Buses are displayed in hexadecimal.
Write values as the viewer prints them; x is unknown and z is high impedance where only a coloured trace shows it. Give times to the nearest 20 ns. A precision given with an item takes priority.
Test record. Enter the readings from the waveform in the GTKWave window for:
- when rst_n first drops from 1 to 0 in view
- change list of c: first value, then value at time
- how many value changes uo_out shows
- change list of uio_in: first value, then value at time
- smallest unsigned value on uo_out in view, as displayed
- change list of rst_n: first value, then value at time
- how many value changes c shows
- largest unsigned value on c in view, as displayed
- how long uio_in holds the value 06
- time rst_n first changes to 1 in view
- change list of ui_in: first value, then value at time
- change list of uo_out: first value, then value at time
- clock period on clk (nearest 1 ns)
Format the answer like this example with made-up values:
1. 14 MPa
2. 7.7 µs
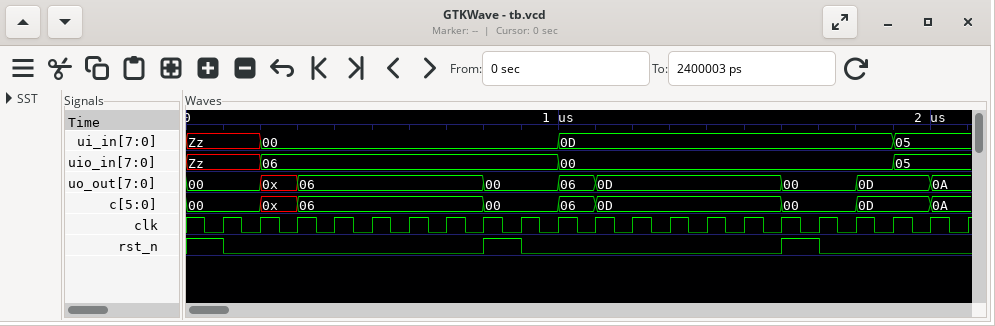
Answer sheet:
1. 100 ns
2. 00, 0x at 200 ns, 06 at 300 ns, 00 at 800 ns, 06 at 1000 ns, 0D at 1100 ns, 00 at 1600 ns, 0D at 1800 ns, 0A at 2000 ns
3. 8
4. Zz, 06 at 200 ns, 00 at 1000 ns, 05 at 1900 ns
5. 00
6. 1, 0 at 100 ns, 1 at 800 ns, 0 at 900 ns, 1 at 1600 ns, 0 at 1700 ns
7. 8
8. 0D
9. 800 ns
10. 800 ns
11. Zz, 00 at 200 ns, 0D at 1000 ns, 05 at 1900 ns
12. 00, 0x at 200 ns, 06 at 300 ns, 00 at 800 ns, 06 at 1000 ns, 0D at 1100 ns, 00 at 1600 ns, 0D at 1800 ns, 0A at 2000 ns
13. 100 ns
